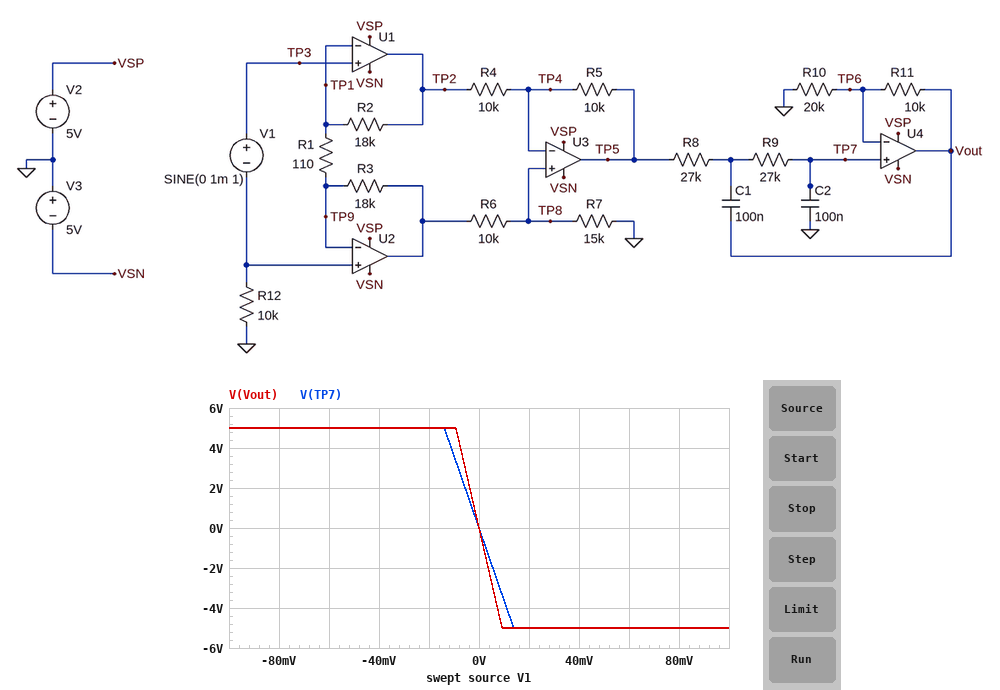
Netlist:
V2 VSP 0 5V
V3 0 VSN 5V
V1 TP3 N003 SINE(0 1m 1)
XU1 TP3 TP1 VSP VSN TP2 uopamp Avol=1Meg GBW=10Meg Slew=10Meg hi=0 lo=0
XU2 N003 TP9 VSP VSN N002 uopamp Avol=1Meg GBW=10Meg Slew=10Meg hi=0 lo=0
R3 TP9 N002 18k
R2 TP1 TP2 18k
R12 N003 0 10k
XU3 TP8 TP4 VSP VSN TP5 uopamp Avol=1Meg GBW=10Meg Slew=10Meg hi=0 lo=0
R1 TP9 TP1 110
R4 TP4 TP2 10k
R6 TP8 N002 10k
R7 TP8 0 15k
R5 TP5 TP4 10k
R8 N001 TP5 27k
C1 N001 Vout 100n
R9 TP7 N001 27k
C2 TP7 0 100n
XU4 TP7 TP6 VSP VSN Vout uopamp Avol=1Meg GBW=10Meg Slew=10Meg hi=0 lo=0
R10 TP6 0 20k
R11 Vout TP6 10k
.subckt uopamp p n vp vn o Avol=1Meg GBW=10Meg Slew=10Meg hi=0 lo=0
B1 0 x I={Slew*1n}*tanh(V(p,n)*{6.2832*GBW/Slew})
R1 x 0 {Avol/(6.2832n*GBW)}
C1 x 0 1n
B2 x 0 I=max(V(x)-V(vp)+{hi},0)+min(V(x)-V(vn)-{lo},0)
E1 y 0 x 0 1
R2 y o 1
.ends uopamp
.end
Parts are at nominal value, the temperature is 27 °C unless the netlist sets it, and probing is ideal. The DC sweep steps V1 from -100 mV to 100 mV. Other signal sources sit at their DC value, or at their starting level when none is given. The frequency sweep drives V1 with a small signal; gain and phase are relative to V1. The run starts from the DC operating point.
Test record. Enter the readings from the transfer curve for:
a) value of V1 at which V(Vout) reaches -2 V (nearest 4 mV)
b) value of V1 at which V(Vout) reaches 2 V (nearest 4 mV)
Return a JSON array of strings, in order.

["4 mV", "-4 mV"]
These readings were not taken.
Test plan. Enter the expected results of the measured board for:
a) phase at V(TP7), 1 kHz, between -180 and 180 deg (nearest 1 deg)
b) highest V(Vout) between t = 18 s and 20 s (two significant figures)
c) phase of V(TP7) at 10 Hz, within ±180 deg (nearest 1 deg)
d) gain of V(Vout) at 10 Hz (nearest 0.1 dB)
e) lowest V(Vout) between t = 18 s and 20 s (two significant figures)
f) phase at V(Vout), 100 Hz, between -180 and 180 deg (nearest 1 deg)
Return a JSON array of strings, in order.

["3 deg", "540 mV", "165 deg", "54.6 dB", "-540 mV", "53 deg"]
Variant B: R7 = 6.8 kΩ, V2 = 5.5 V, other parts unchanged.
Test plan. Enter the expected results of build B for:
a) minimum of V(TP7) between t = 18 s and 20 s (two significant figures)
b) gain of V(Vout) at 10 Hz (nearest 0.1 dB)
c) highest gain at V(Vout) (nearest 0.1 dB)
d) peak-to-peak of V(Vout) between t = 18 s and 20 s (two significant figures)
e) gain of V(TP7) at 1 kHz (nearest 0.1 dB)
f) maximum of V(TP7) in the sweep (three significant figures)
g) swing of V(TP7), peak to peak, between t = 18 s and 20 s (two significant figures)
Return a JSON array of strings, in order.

["-300 mV", "52.9 dB", "53.0 dB", "890 mV", "0.3 dB", "5.51 V", "590 mV"]
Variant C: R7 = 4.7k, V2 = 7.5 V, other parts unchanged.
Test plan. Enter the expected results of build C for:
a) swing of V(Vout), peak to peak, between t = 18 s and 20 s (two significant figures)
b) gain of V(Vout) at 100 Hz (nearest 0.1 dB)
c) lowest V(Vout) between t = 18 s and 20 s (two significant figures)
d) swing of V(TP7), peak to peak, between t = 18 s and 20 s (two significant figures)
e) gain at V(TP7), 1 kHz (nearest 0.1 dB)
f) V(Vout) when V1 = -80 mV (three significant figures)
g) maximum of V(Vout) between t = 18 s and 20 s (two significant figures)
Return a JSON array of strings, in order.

["810 mV", "42.1 dB", "-400 mV", "540 mV", "-0.6 dB", "7.51 V", "400 mV"]
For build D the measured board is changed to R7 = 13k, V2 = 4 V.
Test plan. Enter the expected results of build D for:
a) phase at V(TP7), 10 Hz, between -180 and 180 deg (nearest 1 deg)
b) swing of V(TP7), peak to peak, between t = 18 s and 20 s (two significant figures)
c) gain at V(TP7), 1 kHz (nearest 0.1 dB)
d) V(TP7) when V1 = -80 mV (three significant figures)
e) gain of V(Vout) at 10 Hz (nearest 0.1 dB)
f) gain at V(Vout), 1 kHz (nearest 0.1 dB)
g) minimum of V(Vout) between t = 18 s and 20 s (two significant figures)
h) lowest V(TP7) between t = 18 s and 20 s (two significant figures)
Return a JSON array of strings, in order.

["165 deg", "700 mV", "1.7 dB", "4.01 V", "54.4 dB", "5.2 dB", "-520 mV", "-350 mV"]
